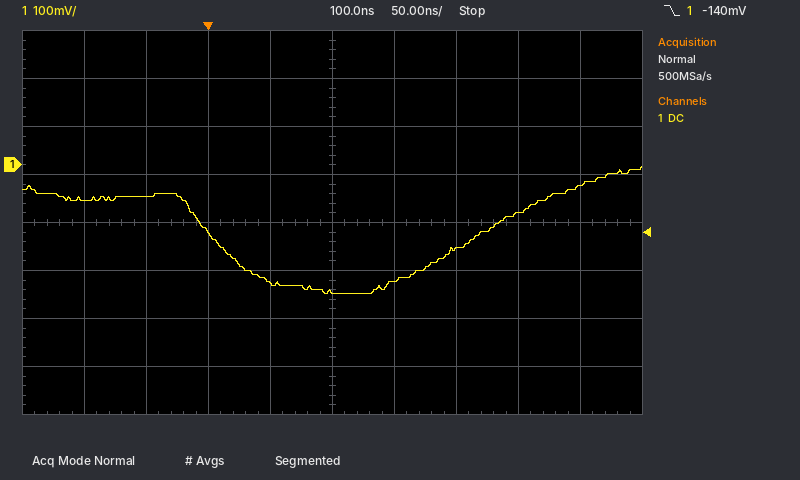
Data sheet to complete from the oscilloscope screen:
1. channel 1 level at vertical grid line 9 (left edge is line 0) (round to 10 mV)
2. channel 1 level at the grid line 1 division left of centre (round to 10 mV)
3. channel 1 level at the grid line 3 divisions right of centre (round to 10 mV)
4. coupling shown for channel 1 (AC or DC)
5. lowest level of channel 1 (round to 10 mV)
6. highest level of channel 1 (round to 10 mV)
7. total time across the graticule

-40 mV
-250 mV
-100 mV
DC
-270 mV
0 mV
500 ns
